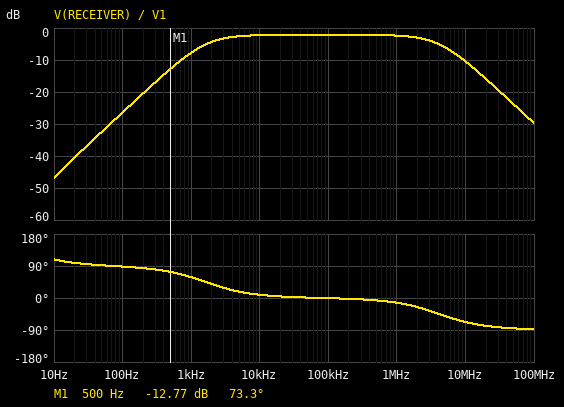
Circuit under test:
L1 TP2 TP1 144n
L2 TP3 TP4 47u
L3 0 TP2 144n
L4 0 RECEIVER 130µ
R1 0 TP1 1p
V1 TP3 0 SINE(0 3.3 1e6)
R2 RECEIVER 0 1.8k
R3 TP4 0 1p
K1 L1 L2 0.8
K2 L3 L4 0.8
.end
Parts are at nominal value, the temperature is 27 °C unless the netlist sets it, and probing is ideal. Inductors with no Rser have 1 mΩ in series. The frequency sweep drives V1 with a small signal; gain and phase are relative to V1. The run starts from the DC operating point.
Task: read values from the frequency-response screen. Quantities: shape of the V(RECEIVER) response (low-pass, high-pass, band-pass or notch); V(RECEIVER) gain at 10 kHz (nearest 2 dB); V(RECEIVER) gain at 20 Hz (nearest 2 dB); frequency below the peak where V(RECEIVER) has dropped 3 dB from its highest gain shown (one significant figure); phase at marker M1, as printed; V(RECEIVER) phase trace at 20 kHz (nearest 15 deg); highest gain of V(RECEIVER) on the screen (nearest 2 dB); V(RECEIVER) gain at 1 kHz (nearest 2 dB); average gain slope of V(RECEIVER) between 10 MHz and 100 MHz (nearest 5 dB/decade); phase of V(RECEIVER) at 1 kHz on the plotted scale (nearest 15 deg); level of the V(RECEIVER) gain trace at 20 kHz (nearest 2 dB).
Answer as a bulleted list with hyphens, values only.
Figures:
- band-pass
- -2 dB
- -40 dB
- 2 kHz
- 73.3 deg
- 0 deg
- -2 dB
- -8 dB
- -20 dB/decade
- 60 deg
- -2 dB
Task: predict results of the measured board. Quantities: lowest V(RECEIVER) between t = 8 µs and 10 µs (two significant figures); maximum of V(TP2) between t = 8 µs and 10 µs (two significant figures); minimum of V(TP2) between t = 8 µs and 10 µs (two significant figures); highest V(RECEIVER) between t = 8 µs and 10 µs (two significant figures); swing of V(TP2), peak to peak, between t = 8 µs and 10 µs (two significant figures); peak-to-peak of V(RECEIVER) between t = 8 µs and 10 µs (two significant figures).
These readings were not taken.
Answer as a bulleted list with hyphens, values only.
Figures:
- -2.5 V
- 110 mV
- -110 mV
- 2.5 V
- 210 mV
- 5.0 V
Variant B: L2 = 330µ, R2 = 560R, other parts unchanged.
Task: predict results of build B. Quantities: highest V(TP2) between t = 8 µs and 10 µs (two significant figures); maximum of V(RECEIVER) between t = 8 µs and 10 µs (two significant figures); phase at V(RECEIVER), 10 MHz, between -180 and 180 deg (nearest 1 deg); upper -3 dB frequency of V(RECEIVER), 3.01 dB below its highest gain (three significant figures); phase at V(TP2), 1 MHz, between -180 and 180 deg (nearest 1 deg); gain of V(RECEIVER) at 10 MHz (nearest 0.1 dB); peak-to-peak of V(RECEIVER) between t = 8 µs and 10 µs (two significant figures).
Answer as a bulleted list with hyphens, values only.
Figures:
- 36 mV
- 770 mV
- -83 deg
- 1.30 MHz
- -10 deg
- -28.4 dB
- 1.5 V
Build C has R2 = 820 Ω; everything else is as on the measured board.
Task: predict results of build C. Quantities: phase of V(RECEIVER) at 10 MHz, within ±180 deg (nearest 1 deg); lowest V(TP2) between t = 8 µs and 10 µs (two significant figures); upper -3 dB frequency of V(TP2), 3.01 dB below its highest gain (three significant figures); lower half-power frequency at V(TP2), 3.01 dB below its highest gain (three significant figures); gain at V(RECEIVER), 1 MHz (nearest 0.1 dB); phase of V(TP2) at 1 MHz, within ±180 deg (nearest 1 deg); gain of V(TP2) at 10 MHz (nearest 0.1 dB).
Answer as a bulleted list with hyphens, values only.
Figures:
- -79 deg
- -100 mV
- 6.97 MHz
- 448 Hz
- -3.2 dB
- -8 deg
- -32.9 dB
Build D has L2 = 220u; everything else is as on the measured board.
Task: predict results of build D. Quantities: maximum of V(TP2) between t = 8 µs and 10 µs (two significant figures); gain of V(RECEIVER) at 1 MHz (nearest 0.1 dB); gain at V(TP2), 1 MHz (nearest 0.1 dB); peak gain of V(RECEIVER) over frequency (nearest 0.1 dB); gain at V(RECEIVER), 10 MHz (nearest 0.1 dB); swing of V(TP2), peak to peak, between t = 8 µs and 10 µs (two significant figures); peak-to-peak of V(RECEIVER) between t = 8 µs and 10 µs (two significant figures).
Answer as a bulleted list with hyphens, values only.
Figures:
- 49 mV
- -9.1 dB
- -36.6 dB
- -8.8 dB
- -17.1 dB
- 98 mV
- 2.3 V
